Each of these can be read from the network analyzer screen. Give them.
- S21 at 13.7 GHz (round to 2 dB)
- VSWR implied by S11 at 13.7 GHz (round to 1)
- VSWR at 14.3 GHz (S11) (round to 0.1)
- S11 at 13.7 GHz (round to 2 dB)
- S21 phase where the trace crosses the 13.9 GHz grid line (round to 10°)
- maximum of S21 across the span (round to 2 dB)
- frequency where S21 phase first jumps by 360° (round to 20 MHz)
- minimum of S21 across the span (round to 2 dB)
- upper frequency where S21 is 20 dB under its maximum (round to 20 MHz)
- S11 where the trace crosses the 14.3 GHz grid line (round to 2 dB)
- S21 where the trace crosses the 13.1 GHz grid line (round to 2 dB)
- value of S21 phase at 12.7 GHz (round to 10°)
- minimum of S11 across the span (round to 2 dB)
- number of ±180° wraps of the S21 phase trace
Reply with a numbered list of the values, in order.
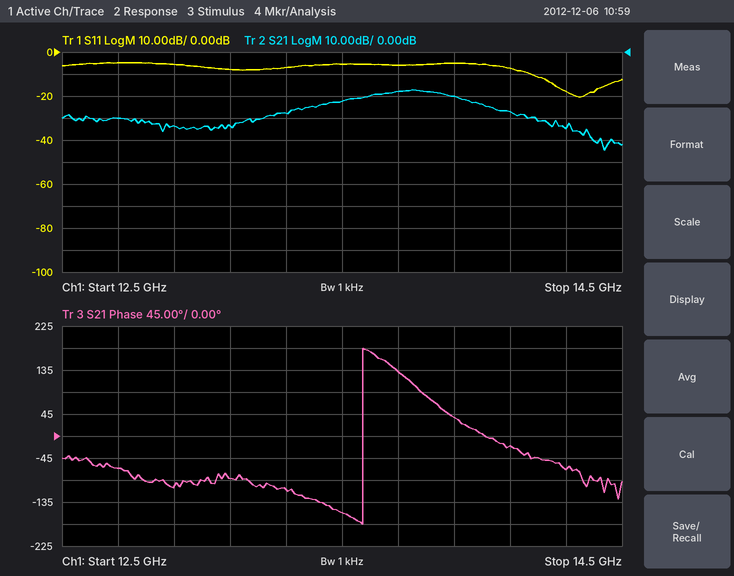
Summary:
1. -18 dB
2. 3
3. 1.3
4. -6 dB
5. 40°
6. -18 dB
7. 13.58 GHz
8. -44 dB
9. 14.36 GHz
10. -18 dB
11. -34 dB
12. -70°
13. -20 dB
14. 1
